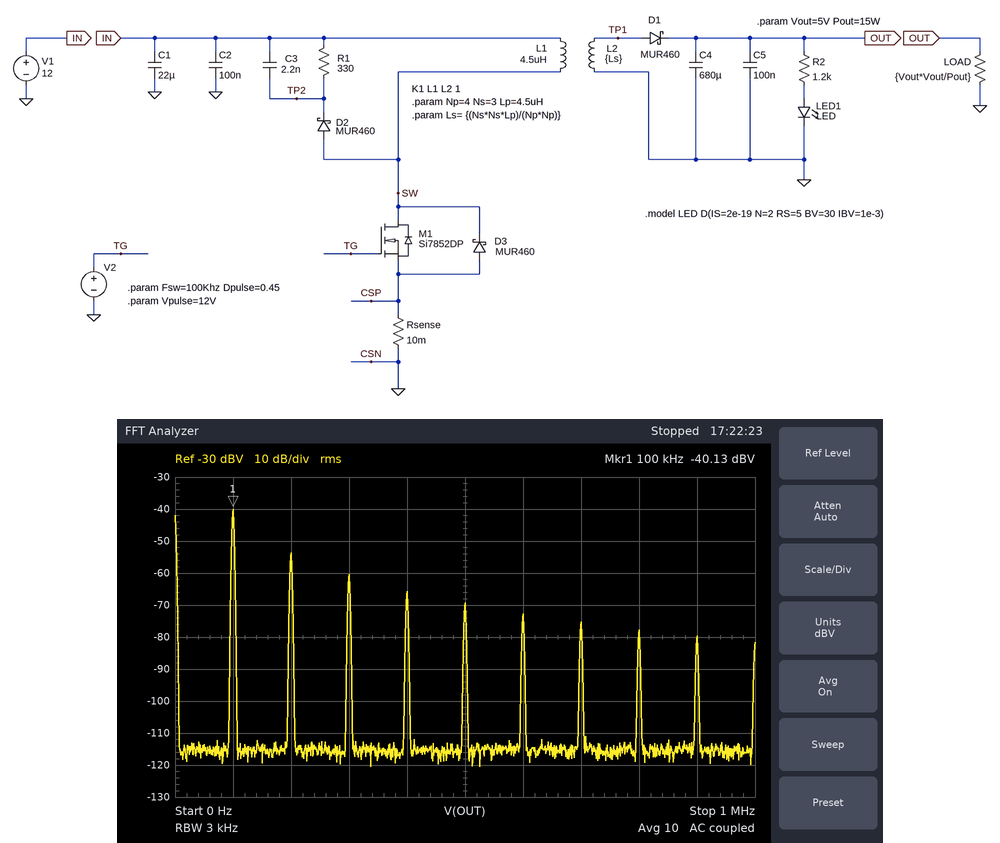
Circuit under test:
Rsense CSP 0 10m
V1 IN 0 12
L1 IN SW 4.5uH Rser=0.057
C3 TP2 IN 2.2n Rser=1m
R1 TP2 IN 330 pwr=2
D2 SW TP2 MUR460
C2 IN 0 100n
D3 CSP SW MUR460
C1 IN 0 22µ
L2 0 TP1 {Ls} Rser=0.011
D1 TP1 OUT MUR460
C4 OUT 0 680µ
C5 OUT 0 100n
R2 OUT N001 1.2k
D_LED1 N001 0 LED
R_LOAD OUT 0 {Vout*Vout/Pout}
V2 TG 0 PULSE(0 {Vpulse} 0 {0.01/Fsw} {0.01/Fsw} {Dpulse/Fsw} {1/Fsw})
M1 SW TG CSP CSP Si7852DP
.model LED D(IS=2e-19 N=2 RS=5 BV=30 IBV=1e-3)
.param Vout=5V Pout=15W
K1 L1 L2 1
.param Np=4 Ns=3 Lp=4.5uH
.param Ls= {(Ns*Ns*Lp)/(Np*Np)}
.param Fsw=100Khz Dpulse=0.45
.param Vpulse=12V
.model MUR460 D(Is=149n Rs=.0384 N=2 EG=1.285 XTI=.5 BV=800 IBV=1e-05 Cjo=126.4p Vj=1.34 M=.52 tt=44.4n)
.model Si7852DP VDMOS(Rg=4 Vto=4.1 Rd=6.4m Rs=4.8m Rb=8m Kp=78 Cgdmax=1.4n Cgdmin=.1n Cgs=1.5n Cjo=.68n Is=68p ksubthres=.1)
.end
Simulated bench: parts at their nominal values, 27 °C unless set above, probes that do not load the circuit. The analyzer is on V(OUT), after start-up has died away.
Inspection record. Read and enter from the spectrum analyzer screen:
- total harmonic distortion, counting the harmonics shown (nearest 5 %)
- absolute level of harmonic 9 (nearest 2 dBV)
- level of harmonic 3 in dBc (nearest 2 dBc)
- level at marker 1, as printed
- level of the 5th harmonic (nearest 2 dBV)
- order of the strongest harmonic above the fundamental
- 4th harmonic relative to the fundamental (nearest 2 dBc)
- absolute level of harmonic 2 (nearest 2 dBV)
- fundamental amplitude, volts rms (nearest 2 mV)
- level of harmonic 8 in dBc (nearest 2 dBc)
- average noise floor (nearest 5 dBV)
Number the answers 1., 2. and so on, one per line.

1. 25 %
2. -80 dBV
3. -20 dBc
4. -40.13 dBV
5. -70 dBV
6. 2
7. -26 dBc
8. -54 dBV
9. 10 mV
10. -38 dBc
11. -115 dBV
